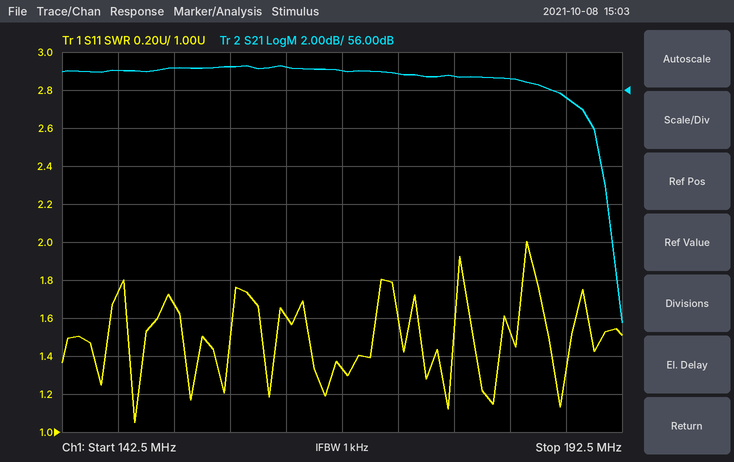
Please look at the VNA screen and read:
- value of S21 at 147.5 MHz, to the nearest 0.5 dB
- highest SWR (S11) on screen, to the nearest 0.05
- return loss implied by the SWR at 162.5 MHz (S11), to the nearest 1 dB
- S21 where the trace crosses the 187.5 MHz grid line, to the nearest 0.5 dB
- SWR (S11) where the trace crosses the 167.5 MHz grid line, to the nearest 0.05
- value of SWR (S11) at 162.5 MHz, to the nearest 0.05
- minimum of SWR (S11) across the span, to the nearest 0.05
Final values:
57.0 dB
2.00
13 dB
55.5 dB
1.35
1.60
1.05
